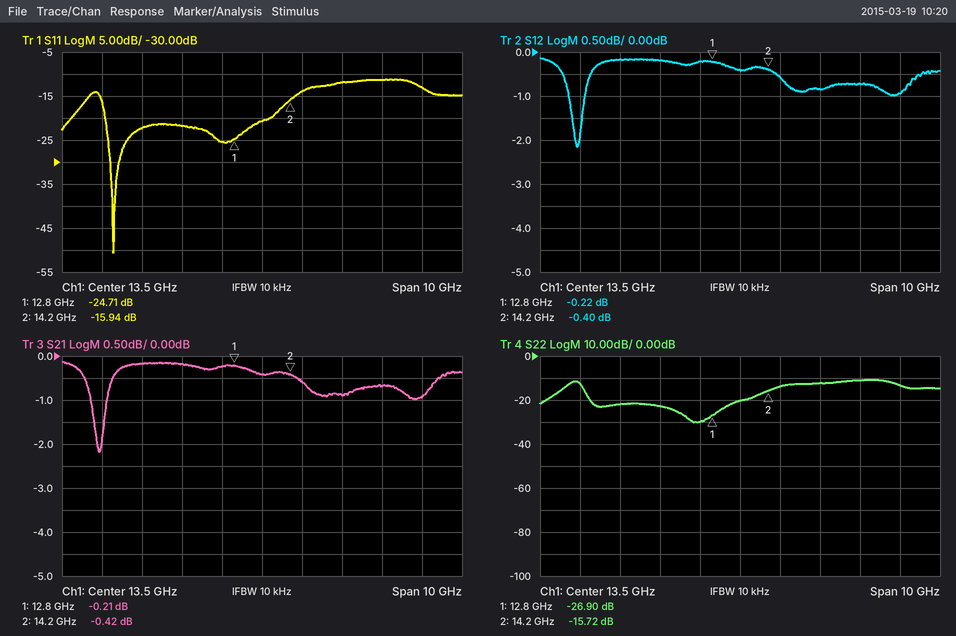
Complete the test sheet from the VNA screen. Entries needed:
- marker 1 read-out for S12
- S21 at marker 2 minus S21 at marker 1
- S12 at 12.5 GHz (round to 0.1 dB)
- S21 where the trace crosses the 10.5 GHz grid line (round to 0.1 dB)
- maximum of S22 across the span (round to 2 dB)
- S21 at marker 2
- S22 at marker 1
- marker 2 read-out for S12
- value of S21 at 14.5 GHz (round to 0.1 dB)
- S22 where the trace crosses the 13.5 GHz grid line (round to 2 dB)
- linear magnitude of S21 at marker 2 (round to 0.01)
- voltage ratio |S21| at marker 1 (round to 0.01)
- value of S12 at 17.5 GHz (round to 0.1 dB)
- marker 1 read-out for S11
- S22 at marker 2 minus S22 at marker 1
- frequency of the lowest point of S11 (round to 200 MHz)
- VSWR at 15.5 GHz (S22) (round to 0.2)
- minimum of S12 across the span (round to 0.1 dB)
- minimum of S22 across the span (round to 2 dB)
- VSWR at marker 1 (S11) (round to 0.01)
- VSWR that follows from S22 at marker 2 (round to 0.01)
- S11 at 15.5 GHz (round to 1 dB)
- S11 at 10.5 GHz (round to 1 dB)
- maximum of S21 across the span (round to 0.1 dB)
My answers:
-0.22 dB
-0.21 dB
-0.2 dB
-0.2 dB
-10 dB
-0.42 dB
-26.90 dB
-0.40 dB
-0.6 dB
-20 dB
0.95
0.98
-0.9 dB
-24.71 dB
11.18 dB
9.8 GHz
1.6
-2.2 dB
-30 dB
1.12
1.39
-12 dB
-22 dB
-0.1 dB
